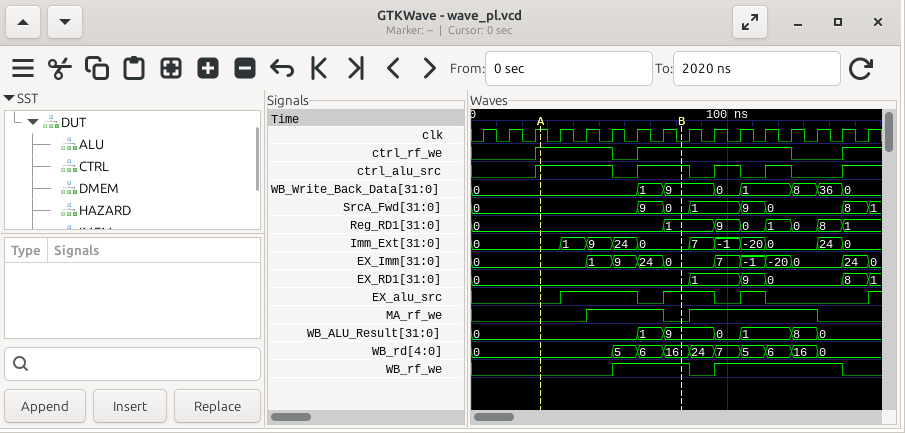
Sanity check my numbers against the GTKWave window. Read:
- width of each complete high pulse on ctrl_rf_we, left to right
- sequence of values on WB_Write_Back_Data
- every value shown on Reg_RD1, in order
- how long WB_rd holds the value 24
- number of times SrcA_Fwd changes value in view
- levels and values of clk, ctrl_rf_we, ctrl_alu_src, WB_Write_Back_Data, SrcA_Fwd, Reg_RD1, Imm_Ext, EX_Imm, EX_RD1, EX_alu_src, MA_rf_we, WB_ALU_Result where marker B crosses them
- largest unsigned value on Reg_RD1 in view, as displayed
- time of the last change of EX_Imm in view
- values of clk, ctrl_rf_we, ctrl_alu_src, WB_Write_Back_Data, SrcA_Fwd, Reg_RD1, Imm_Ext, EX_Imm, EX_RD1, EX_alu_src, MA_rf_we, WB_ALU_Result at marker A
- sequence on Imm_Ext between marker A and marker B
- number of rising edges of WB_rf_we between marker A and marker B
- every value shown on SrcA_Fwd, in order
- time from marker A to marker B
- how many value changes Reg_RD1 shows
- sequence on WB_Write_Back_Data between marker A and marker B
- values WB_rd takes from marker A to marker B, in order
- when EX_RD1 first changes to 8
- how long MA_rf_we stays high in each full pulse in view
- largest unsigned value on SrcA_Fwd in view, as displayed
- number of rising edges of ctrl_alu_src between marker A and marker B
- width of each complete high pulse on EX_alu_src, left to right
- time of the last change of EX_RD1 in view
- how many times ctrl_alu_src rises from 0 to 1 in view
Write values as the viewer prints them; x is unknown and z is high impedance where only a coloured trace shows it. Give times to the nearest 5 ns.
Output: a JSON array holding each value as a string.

["30 ns, 60 ns", "0, 1, 9, 0, 1, 8, 36, 0", "0, 1, 9, 0, 1, 0, 8, 1", "10 ns", "7", "clk=0, ctrl_rf_we=1, ctrl_alu_src=1, WB_Write_Back_Data=9, SrcA_Fwd=0, Reg_RD1=1, Imm_Ext=0, EX_Imm=0, EX_RD1=0, EX_alu_src=1, MA_rf_we=0, WB_ALU_Result=9", "9", "155 ns", "clk=1, ctrl_rf_we=1, ctrl_alu_src=1, WB_Write_Back_Data=0, SrcA_Fwd=0, Reg_RD1=0, Imm_Ext=0, EX_Imm=0, EX_RD1=0, EX_alu_src=0, MA_rf_we=0, WB_ALU_Result=0", "0, 1, 9, 24, 0", "1", "0, 9, 0, 1, 9, 0, 8, 1", "55 ns", "7", "0, 1, 9", "0, 5, 6, 16", "145 ns", "30 ns, 50 ns", "9", "1", "30 ns, 20 ns, 10 ns", "155 ns", "5"]
